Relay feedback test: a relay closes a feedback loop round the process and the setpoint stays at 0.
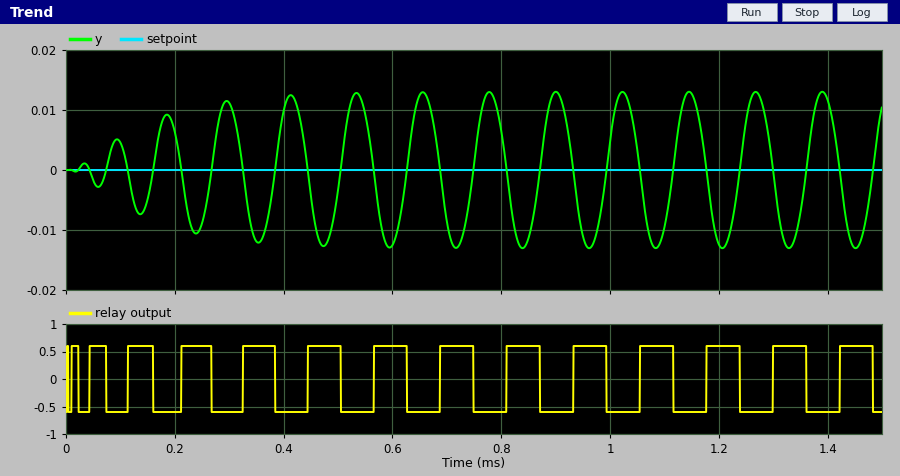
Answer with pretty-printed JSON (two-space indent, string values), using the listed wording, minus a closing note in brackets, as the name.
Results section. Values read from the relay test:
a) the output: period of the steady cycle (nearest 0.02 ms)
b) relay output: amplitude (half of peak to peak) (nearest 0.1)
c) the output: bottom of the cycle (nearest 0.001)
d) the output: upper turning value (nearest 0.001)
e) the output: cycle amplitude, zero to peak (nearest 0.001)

{
  "the output: period of the steady cycle": "0.12 ms",
  "relay output: amplitude (half of peak to peak)": "0.6",
  "the output: bottom of the cycle": "-0.013",
  "the output: upper turning value": "0.013",
  "the output: cycle amplitude, zero to peak": "0.013"
}
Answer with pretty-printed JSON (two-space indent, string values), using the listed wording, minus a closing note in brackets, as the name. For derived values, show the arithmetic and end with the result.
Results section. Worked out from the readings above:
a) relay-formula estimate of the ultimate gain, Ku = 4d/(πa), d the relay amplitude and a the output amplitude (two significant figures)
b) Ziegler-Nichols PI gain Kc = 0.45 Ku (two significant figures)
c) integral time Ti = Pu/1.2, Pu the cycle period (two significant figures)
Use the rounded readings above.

{
  "relay-formula estimate of the ultimate gain, Ku = 4d/(πa), d the relay amplitude and a the output amplitude": "4 × 0.6 / (π × 0.013) = 59",
  "Ziegler-Nichols PI gain Kc = 0.45 Ku": "0.45 × 59 = 27",
  "integral time Ti = Pu/1.2, Pu the cycle period": "0.12 / 1.2 = 0.10 ms"
}
